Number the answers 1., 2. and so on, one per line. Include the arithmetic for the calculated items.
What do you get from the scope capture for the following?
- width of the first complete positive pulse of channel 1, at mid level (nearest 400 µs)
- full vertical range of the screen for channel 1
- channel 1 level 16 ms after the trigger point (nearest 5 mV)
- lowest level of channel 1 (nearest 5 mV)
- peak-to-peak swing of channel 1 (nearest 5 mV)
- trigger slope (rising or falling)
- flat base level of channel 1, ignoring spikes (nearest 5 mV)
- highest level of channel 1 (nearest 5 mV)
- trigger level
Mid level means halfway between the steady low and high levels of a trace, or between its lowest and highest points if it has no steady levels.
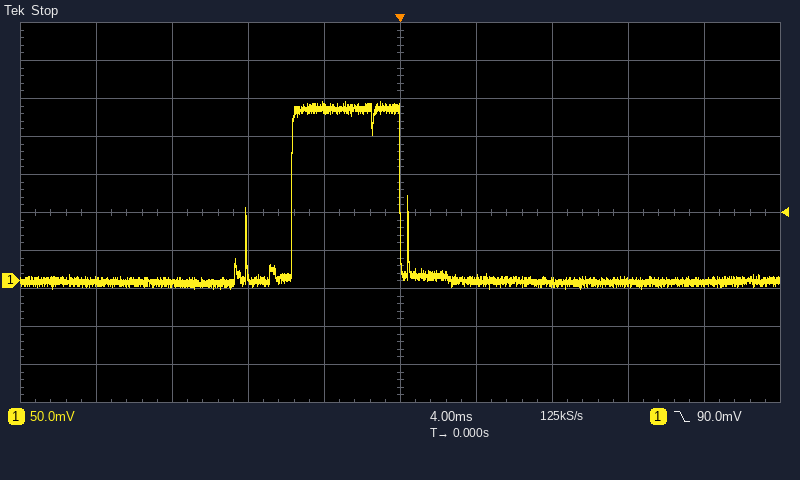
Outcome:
1. 5.6 ms
2. 500 mV
3. 0 mV
4. -10 mV
5. 235 mV − (-10 mV) = 245 mV
6. falling
7. 0 mV
8. 235 mV
9. 90.0 mV
